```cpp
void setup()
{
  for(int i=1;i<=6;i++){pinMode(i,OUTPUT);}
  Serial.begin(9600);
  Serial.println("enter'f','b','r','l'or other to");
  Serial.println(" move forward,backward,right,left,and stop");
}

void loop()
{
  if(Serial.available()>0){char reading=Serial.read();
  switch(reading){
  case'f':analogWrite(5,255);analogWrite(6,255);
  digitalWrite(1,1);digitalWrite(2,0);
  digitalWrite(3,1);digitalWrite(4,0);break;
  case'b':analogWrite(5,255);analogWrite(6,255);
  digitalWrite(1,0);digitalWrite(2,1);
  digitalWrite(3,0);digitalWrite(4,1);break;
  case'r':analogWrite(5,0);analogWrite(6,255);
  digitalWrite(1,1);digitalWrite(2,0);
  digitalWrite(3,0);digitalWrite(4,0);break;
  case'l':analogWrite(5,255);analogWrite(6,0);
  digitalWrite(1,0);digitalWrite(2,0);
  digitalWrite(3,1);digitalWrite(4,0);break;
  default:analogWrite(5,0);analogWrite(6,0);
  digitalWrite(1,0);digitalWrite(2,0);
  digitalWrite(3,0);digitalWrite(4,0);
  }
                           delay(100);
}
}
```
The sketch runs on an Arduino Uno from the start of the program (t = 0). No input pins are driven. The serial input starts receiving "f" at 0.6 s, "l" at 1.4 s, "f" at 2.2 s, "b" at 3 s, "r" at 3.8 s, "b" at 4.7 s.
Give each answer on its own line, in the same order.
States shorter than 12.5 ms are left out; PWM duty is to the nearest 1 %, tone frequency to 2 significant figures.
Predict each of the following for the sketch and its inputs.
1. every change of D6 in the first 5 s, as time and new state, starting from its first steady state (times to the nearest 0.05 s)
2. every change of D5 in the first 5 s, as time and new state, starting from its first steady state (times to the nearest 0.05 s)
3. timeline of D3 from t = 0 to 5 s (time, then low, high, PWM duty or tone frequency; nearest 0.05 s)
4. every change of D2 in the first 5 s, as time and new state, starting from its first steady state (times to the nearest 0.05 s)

0 s low; 0.6 s high; 1.4 s low; 2.2 s high
0 s low; 0.6 s high; 3.8 s low; 4.7 s high
0 s low; 0.6 s high; 3 s low
0 s low; 3 s high; 3.8 s low; 4.7 s high
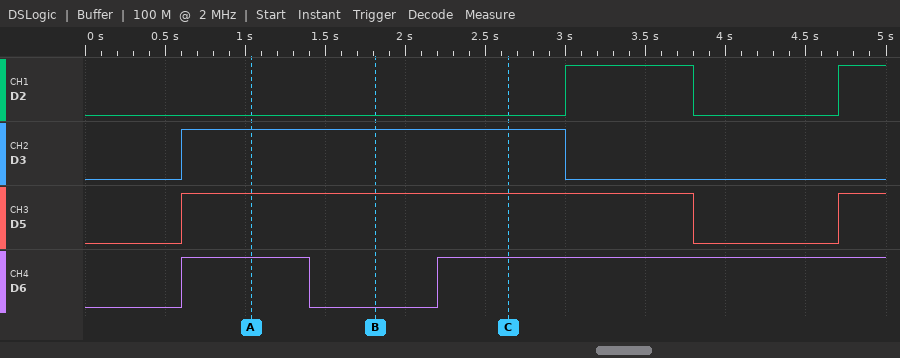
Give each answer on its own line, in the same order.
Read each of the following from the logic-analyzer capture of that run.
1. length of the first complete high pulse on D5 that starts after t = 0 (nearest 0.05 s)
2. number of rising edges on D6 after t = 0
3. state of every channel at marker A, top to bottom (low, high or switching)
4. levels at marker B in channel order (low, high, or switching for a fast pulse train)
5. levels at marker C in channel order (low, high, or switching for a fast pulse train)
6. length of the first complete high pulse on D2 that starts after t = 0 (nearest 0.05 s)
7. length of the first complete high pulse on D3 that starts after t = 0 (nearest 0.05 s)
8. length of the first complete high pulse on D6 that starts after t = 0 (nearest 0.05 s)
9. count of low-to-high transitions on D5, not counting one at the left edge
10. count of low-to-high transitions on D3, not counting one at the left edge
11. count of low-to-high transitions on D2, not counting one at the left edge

3.20 s
2
D2 low, D3 high, D5 high, D6 high
D2 low, D3 high, D5 high, D6 low
D2 low, D3 high, D5 high, D6 high
0.80 s
2.40 s
0.80 s
2
1
2
